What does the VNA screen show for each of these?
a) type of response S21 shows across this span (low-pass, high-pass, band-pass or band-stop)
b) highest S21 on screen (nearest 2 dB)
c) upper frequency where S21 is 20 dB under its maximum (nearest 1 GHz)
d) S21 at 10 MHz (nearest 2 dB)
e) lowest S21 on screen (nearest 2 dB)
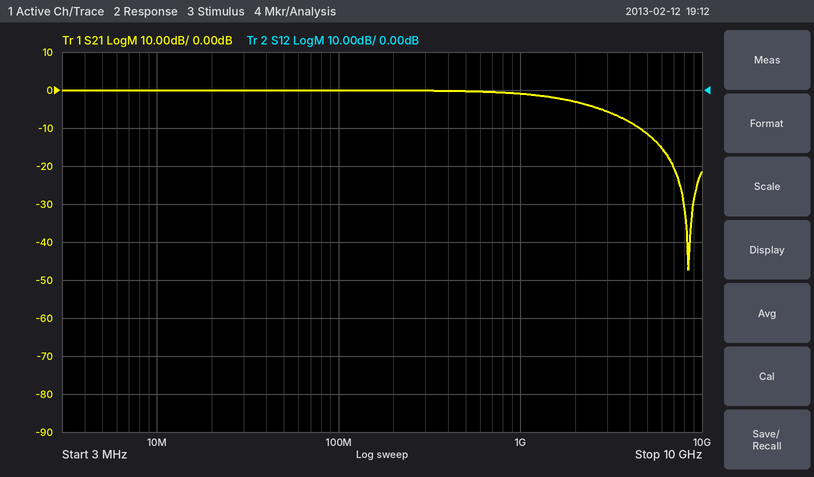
low-pass
0 dB
7 GHz
0 dB
-48 dB
